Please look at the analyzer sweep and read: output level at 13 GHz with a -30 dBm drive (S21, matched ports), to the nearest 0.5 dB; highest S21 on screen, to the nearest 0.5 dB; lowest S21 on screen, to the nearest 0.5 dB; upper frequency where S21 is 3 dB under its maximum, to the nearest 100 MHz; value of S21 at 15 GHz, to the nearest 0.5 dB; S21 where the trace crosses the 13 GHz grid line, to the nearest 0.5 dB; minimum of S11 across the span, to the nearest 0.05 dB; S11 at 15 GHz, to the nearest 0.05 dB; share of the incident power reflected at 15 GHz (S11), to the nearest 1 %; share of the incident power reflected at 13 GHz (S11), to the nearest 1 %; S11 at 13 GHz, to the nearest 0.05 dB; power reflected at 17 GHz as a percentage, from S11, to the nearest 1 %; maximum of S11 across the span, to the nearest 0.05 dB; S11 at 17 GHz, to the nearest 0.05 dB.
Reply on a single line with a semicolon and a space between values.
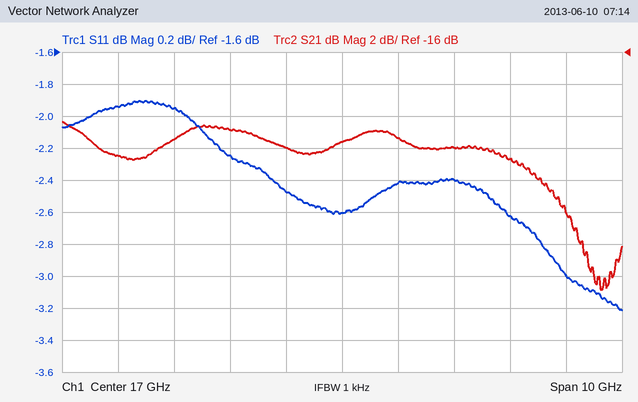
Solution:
-52.5 dBm; -20.5 dB; -31.0 dB; 20.3 GHz; -21.0 dB; -22.5 dB; -3.20 dB; -2.25 dB; 60 %; 64 %; -1.95 dB; 55 %; -1.90 dB; -2.60 dB
